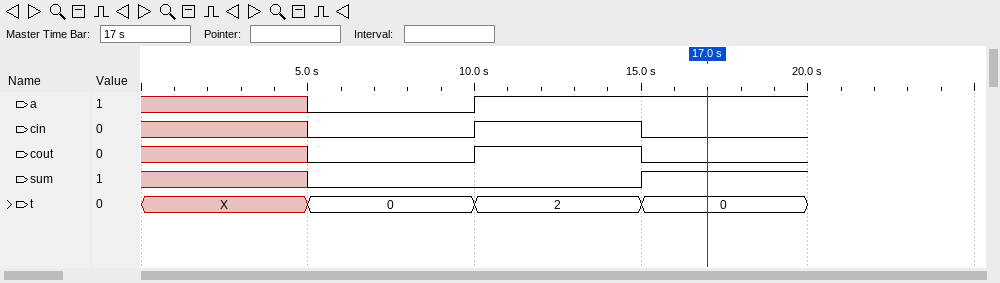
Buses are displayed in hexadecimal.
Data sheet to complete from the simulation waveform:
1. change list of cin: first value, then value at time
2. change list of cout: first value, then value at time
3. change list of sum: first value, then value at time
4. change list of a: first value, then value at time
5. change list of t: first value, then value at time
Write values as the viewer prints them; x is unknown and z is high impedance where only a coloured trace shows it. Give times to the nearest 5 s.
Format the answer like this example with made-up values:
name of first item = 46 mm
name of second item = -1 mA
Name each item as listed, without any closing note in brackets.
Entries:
change list of cin: first value, then value at time = x, 0 at 5 s, 1 at 10 s, 0 at 15 s
change list of cout: first value, then value at time = x, 0 at 5 s, 1 at 10 s, 0 at 15 s
change list of sum: first value, then value at time = x, 0 at 5 s, 1 at 15 s
change list of a: first value, then value at time = x, 0 at 5 s, 1 at 10 s
change list of t: first value, then value at time = X, 0 at 5 s, 2 at 10 s, 0 at 15 s
